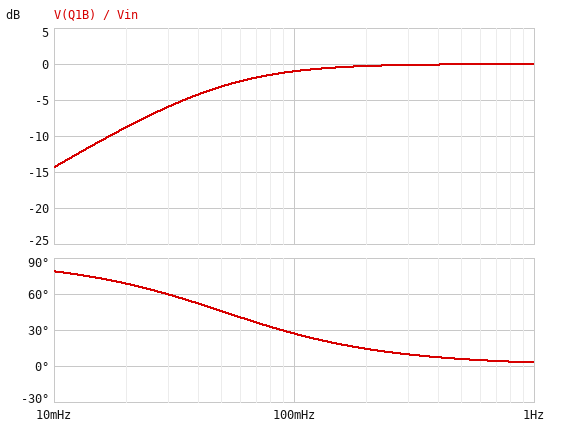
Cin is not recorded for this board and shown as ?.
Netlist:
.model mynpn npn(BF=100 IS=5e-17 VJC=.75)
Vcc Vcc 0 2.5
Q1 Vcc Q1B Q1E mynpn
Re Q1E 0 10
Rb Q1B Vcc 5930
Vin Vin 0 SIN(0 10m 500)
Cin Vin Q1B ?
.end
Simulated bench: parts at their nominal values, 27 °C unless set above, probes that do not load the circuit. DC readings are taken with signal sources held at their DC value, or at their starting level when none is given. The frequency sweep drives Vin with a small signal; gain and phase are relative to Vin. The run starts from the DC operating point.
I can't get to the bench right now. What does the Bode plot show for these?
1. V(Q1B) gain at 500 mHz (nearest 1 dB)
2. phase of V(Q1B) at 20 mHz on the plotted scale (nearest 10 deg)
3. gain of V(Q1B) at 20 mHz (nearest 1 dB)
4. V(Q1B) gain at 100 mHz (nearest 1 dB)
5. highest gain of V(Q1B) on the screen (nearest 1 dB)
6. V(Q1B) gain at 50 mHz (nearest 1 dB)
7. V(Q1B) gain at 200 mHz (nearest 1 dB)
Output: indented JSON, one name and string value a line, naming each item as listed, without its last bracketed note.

{
  "V(Q1B) gain at 500 mHz": "0 dB",
  "phase of V(Q1B) at 20 mHz on the plotted scale": "70 deg",
  "gain of V(Q1B) at 20 mHz": "-9 dB",
  "V(Q1B) gain at 100 mHz": "-1 dB",
  "highest gain of V(Q1B) on the screen": "0 dB",
  "V(Q1B) gain at 50 mHz": "-3 dB",
  "V(Q1B) gain at 200 mHz": "0 dB"
}
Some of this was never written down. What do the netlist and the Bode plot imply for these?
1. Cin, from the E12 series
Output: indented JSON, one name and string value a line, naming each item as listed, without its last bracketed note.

{
  "Cin, from the E12 series": "3.3 mF"
}
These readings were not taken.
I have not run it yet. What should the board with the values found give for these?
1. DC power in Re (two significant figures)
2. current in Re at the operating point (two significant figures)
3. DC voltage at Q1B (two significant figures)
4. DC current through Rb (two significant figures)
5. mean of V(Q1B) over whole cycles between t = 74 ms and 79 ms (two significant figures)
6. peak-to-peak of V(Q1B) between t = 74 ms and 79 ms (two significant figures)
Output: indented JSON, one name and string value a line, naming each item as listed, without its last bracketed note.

{
  "DC power in Re": "5.6 mW",
  "current in Re at the operating point": "24 mA",
  "DC voltage at Q1B": "1.1 V",
  "DC current through Rb": "230 µA",
  "mean of V(Q1B) over whole cycles between t = 74 ms and 79 ms": "1.1 V",
  "peak-to-peak of V(Q1B) between t = 74 ms and 79 ms": "20 mV"
}
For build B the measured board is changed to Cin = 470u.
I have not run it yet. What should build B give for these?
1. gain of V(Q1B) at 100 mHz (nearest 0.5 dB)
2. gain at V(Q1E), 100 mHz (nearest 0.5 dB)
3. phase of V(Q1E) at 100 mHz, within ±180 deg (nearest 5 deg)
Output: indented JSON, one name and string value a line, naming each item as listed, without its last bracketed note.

{
  "gain of V(Q1B) at 100 mHz": "-11.5 dB",
  "gain at V(Q1E), 100 mHz": "-12.5 dB",
  "phase of V(Q1E) at 100 mHz, within ±180 deg": "75 deg"
}
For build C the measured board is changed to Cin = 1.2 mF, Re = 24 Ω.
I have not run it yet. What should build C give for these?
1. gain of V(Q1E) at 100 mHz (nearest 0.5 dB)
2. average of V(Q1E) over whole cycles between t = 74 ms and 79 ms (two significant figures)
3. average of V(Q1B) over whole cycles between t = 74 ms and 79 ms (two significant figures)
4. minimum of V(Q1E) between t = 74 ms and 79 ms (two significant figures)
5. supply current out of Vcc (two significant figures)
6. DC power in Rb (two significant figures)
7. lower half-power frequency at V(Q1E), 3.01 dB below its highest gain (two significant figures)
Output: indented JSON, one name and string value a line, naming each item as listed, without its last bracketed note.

{
  "gain of V(Q1E) at 100 mHz": "-2.5 dB",
  "average of V(Q1E) over whole cycles between t = 74 ms and 79 ms": "470 mV",
  "average of V(Q1B) over whole cycles between t = 74 ms and 79 ms": "1.3 V",
  "minimum of V(Q1E) between t = 74 ms and 79 ms": "460 mV",
  "supply current out of Vcc": "20 mA",
  "DC power in Rb": "230 µW",
  "lower half-power frequency at V(Q1E), 3.01 dB below its highest gain": "74 mHz"
}
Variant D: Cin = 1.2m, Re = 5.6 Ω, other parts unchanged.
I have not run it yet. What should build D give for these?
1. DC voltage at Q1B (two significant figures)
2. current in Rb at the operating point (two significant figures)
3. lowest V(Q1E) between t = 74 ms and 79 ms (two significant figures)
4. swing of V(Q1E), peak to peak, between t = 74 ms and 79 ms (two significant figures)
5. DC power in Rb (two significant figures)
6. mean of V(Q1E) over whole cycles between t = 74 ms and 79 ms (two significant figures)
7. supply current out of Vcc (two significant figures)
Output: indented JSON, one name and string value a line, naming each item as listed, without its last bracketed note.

{
  "DC voltage at Q1B": "1.0 V",
  "current in Rb at the operating point": "250 µA",
  "lowest V(Q1E) between t = 74 ms and 79 ms": "130 mV",
  "swing of V(Q1E), peak to peak, between t = 74 ms and 79 ms": "17 mV",
  "DC power in Rb": "370 µW",
  "mean of V(Q1E) over whole cycles between t = 74 ms and 79 ms": "140 mV",
  "supply current out of Vcc": "25 mA"
}
